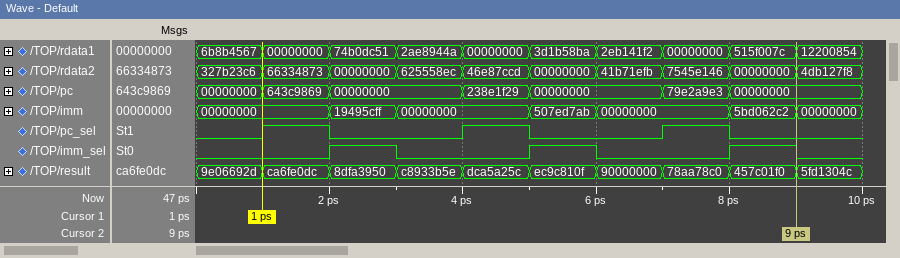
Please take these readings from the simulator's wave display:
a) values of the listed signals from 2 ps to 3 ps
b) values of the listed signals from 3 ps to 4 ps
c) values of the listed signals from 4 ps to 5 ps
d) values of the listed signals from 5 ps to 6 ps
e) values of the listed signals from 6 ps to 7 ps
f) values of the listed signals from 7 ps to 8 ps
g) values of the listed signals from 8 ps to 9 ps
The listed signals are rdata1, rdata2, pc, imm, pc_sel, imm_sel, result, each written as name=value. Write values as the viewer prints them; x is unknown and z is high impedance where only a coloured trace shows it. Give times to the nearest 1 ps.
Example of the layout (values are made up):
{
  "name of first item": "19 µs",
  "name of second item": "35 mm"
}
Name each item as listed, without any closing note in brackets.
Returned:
{
  "values of the listed signals from 2 ps to 3 ps": "rdata1=74b0dc51, rdata2=00000000, pc=00000000, imm=19495cff, pc_sel=0, imm_sel=1, result=8dfa3950",
  "values of the listed signals from 3 ps to 4 ps": "rdata1=2ae8944a, rdata2=625558ec, pc=00000000, imm=00000000, pc_sel=0, imm_sel=0, result=c8933b5e",
  "values of the listed signals from 4 ps to 5 ps": "rdata1=00000000, rdata2=46e87ccd, pc=238e1f29, imm=00000000, pc_sel=1, imm_sel=0, result=dca5a25c",
  "values of the listed signals from 5 ps to 6 ps": "rdata1=3d1b58ba, rdata2=00000000, pc=00000000, imm=507ed7ab, pc_sel=0, imm_sel=1, result=ec9c810f",
  "values of the listed signals from 6 ps to 7 ps": "rdata1=2eb141f2, rdata2=41b71efb, pc=00000000, imm=00000000, pc_sel=0, imm_sel=0, result=90000000",
  "values of the listed signals from 7 ps to 8 ps": "rdata1=00000000, rdata2=7545e146, pc=79e2a9e3, imm=00000000, pc_sel=1, imm_sel=0, result=78aa78c0",
  "values of the listed signals from 8 ps to 9 ps": "rdata1=515f007c, rdata2=00000000, pc=00000000, imm=5bd062c2, pc_sel=0, imm_sel=1, result=457c01f0"
}
